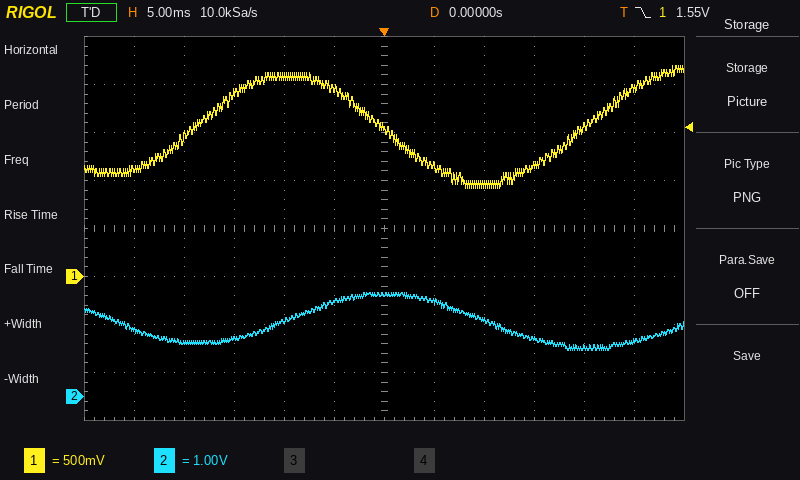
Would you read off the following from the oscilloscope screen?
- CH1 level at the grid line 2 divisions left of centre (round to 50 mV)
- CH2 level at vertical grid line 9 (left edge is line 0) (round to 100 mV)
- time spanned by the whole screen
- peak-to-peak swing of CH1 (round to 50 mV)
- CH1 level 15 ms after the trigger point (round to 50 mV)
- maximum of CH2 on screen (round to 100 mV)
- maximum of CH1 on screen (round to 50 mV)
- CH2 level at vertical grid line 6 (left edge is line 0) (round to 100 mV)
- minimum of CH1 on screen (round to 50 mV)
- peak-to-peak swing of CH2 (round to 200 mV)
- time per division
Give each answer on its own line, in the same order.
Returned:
2.10 V
1.2 V
60 ms
1.30 V
1.15 V
2.2 V
2.20 V
2.1 V
900 mV
1.2 V
5 ms
